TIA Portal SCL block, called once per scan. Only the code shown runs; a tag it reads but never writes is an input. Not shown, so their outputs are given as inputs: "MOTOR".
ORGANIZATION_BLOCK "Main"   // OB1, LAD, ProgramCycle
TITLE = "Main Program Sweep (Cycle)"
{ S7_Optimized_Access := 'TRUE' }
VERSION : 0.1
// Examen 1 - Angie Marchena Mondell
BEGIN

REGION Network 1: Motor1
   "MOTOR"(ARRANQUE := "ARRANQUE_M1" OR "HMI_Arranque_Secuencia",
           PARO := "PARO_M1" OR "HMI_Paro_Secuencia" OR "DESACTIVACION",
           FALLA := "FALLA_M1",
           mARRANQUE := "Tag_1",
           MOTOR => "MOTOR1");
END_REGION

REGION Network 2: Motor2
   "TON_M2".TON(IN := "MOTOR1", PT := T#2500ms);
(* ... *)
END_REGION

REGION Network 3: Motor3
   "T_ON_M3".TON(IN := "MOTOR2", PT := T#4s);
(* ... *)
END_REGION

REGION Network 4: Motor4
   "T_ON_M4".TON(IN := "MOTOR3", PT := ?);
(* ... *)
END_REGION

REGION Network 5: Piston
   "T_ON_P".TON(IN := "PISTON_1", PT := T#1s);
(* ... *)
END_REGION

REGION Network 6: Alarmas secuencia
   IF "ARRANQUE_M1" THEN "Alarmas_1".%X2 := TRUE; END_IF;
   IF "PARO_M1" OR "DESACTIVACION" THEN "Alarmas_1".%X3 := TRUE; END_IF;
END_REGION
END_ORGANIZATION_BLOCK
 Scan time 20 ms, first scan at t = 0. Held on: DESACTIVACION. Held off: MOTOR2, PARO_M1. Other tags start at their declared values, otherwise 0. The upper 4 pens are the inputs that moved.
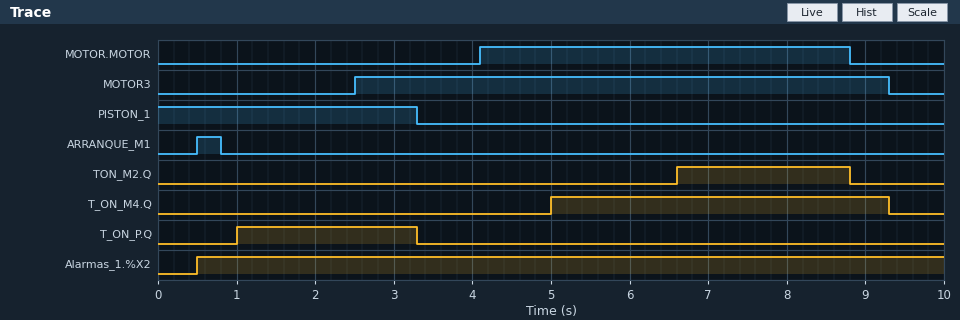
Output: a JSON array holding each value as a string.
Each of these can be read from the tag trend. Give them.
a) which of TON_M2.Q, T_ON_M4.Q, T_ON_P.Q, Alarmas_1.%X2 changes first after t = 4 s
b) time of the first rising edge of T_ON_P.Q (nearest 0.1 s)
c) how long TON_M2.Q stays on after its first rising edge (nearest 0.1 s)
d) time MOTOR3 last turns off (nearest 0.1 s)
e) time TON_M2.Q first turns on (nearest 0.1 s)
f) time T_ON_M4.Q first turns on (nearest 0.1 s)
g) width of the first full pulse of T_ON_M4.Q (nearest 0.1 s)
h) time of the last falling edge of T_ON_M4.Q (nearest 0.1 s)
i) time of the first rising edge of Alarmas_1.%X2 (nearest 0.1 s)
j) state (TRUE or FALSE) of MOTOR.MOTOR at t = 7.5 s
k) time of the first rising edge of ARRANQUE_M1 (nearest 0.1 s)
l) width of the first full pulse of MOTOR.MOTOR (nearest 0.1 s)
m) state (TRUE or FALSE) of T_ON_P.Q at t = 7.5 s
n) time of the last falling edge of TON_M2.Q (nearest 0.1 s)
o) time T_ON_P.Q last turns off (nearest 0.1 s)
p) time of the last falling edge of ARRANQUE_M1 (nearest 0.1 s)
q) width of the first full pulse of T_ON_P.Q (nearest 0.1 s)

["T_ON_M4.Q", "1.0 s", "2.2 s", "9.3 s", "6.6 s", "5.0 s", "4.3 s", "9.3 s", "0.5 s", "TRUE", "0.5 s", "4.7 s", "FALSE", "8.8 s", "3.3 s", "0.8 s", "2.3 s"]
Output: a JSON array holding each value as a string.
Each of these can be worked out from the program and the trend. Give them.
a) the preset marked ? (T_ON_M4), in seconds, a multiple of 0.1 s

["2.5 s"]
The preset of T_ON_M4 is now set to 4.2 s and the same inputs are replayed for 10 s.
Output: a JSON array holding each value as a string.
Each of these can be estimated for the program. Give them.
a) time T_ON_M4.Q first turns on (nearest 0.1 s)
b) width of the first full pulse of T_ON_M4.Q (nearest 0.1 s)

["6.7 s", "2.6 s"]
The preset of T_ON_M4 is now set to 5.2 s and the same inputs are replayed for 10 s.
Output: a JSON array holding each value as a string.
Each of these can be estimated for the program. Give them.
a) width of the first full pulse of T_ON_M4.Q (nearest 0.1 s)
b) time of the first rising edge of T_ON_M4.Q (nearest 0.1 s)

["1.6 s", "7.7 s"]
